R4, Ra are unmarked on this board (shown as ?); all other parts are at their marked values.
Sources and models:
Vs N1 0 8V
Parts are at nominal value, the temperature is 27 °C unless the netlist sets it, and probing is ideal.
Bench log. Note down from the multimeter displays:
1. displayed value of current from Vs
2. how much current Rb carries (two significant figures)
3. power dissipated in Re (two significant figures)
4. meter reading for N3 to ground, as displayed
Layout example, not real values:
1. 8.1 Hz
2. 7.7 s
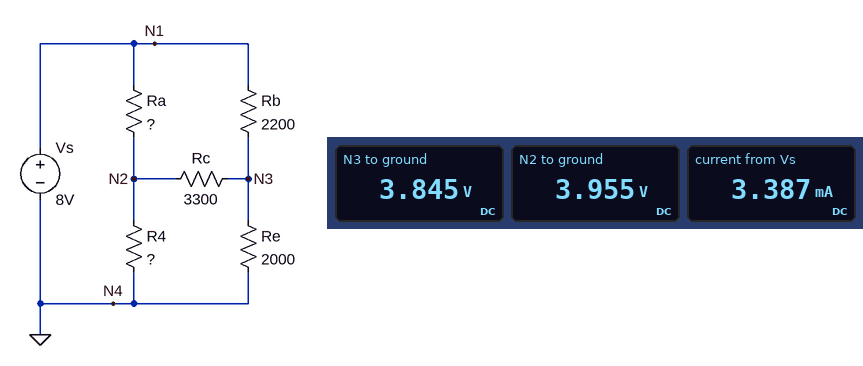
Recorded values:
1. 3.387 mA
2. 1.9 mA
3. 7.4 mW
4. 3.845 V
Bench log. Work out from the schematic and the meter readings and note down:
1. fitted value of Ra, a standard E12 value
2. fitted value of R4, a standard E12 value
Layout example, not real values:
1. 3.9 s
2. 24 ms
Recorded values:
1. 2.7 kΩ
2. 2.7 kΩ
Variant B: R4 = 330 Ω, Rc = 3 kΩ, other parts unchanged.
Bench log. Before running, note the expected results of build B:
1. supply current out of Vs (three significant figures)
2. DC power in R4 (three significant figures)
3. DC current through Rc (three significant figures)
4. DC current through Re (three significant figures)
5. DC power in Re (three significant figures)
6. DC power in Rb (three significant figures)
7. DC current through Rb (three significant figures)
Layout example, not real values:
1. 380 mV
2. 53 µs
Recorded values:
1. 4.79 mA
2. 3.47 mW
3. 677 µA
4. 1.55 mA
5. 4.81 mW
6. 10.9 mW
7. 2.23 mA
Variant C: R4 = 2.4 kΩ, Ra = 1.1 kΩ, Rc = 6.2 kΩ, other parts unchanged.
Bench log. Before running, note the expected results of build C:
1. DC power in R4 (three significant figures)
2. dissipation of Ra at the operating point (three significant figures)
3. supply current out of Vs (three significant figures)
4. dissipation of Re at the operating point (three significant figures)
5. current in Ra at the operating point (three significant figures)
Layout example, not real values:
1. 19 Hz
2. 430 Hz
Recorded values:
1. 11.8 mW
2. 6.49 mW
3. 4.23 mA
4. 8.12 mW
5. 2.43 mA
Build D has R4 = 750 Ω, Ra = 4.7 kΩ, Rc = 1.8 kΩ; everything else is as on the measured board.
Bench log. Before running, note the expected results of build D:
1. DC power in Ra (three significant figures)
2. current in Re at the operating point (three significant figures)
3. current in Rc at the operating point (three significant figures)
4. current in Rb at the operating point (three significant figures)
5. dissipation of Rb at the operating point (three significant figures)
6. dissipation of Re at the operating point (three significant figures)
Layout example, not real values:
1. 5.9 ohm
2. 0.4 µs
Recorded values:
1. 8.71 mW
2. 1.50 mA
3. 775 µA
4. 2.27 mA
5. 11.4 mW
6. 4.49 mW
